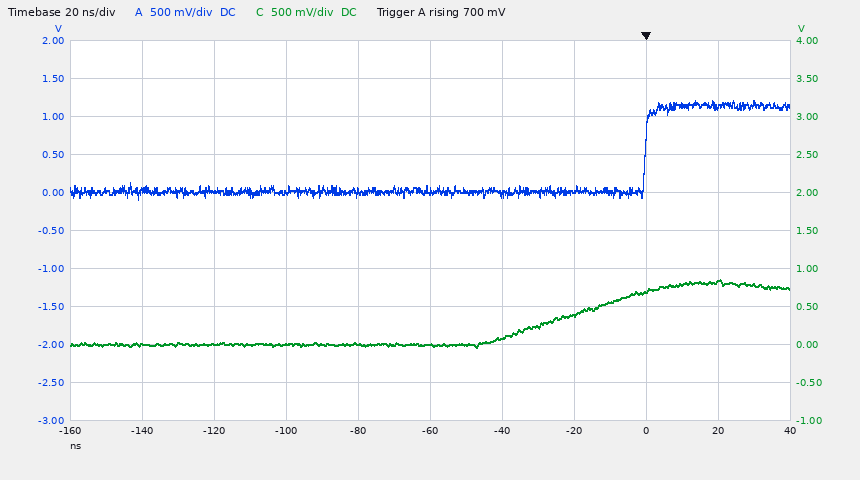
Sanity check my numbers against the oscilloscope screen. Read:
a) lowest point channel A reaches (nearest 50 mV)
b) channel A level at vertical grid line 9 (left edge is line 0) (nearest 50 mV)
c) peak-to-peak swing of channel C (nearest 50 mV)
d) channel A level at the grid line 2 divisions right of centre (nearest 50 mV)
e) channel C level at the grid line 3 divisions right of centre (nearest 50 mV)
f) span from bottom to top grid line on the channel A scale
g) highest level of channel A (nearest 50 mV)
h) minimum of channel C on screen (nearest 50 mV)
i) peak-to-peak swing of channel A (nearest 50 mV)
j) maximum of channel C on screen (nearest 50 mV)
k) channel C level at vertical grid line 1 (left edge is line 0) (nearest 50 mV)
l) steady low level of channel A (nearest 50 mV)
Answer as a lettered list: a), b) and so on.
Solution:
a) -100 mV
b) 1.10 V
c) 900 mV
d) 50 mV
e) 700 mV
f) 5 V
g) 1.20 V
h) -50 mV
i) 1.30 V
j) 850 mV
k) 0 mV
l) 0 mV
